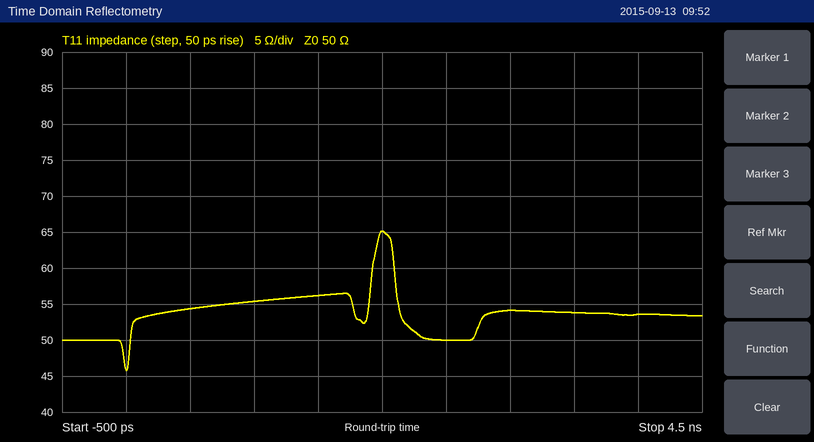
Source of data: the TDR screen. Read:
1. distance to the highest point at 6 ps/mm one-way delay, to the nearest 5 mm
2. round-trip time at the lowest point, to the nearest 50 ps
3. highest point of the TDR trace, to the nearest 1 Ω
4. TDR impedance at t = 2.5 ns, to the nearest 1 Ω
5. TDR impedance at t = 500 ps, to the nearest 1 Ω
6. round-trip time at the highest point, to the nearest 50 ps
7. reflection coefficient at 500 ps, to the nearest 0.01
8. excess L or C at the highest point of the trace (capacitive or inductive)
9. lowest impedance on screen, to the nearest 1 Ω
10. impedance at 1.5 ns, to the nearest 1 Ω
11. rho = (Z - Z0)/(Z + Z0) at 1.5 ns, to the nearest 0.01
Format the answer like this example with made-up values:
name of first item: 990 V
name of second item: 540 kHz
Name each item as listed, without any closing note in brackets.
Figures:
distance to the highest point at 6 ps/mm one-way delay, to the nearest 5 mm: 165 mm
round-trip time at the lowest point, to the nearest 50 ps: 0 ps
highest point of the TDR trace, to the nearest 1 Ω: 65 Ω
TDR impedance at t = 2.5 ns, to the nearest 1 Ω: 50 Ω
TDR impedance at t = 500 ps, to the nearest 1 Ω: 54 Ω
round-trip time at the highest point, to the nearest 50 ps: 2.00 ns
reflection coefficient at 500 ps, to the nearest 0.01: +0.04
excess L or C at the highest point of the trace: inductive
lowest impedance on screen, to the nearest 1 Ω: 46 Ω
impedance at 1.5 ns, to the nearest 1 Ω: 56 Ω
rho = (Z - Z0)/(Z + Z0) at 1.5 ns, to the nearest 0.01: +0.06
